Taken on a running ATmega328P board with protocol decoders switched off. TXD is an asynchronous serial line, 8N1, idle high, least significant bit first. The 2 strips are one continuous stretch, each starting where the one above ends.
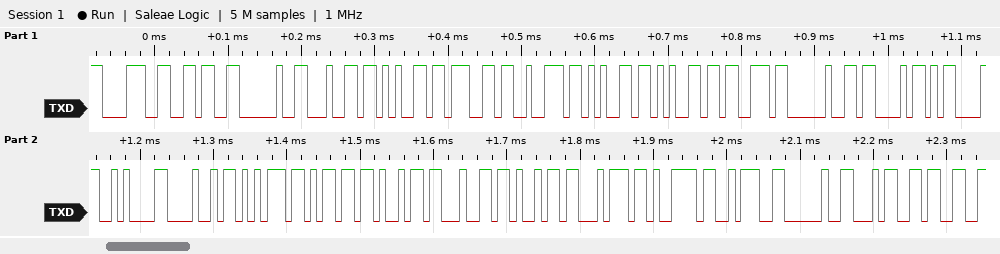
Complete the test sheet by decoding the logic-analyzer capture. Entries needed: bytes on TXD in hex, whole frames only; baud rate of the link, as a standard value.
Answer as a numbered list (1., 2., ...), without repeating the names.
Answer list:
1. 38 36 20 64 65 67 72 65 65 73 20 43 0D 0A 48 75 6D 69 64 69 74 79 3A 20 34 33
2. 115200 baud
